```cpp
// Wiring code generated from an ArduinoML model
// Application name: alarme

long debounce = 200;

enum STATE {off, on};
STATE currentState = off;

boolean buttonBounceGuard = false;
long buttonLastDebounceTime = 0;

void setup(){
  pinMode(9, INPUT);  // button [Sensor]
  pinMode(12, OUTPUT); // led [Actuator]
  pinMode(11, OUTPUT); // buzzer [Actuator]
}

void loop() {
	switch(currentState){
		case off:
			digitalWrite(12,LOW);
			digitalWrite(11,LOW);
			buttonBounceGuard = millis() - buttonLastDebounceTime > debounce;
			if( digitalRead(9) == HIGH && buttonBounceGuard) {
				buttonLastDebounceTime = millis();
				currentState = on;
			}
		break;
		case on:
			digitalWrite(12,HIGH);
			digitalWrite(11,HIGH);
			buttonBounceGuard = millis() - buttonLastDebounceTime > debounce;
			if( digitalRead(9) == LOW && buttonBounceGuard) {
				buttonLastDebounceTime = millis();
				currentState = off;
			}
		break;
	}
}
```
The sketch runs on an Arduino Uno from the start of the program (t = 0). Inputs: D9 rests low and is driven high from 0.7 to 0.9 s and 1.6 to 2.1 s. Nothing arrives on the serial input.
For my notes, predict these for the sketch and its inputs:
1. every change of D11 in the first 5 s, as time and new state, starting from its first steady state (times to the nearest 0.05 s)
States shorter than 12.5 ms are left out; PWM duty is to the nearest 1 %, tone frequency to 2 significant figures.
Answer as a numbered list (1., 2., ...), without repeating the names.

1. 0 s low; 0.7 s high; 0.9 s low; 1.6 s high; 2.1 s low
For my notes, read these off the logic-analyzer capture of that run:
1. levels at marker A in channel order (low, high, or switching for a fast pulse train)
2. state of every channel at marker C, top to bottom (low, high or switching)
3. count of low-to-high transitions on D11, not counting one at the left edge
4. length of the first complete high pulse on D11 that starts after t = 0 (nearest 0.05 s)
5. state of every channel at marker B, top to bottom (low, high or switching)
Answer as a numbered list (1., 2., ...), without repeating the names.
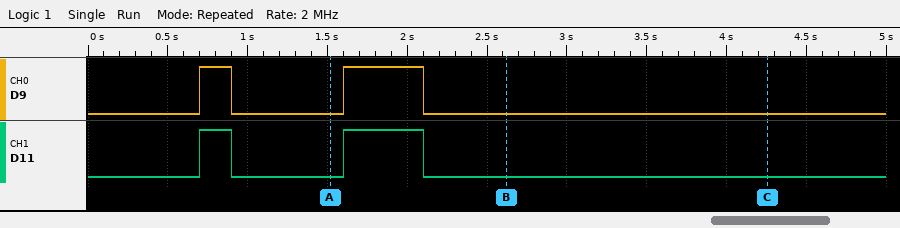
1. D9 low, D11 low
2. D9 low, D11 low
3. 2
4. 0.20 s
5. D9 low, D11 low
